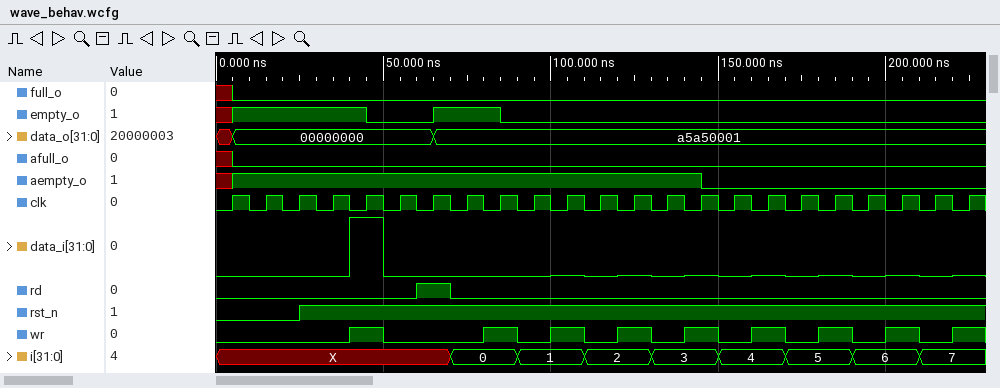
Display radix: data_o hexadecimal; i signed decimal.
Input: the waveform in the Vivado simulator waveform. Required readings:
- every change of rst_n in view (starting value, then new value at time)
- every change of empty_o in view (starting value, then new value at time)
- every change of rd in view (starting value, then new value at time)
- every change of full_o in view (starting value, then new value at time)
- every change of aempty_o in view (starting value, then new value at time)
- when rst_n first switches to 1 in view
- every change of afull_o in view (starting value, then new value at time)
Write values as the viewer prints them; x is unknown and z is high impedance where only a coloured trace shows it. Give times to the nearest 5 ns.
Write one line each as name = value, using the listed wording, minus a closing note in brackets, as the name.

every change of rst_n in view = 0, 1 at 25 ns
every change of empty_o in view = x, 1 at 5 ns, 0 at 45 ns, 1 at 65 ns, 0 at 85 ns
every change of rd in view = 0, 1 at 60 ns, 0 at 70 ns
every change of full_o in view = x, 0 at 5 ns
every change of aempty_o in view = x, 1 at 5 ns, 0 at 145 ns
when rst_n first switches to 1 in view = 25 ns
every change of afull_o in view = x, 0 at 5 ns
